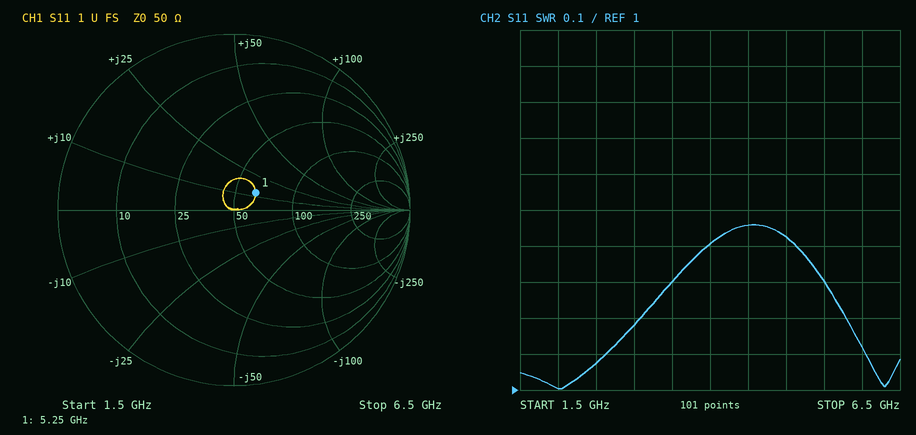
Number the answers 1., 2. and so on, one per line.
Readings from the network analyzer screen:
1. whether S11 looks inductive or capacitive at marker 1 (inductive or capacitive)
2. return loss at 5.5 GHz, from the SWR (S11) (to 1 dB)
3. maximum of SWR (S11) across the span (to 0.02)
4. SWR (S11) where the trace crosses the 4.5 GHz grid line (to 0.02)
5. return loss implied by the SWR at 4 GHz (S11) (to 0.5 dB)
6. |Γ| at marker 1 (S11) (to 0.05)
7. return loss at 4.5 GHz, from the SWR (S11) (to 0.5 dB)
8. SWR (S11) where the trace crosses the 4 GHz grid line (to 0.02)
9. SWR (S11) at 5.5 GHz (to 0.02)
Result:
1. inductive
2. 18 dB
3. 1.46
4. 1.46
5. 15.5 dB
6. 0.15
7. 14.5 dB
8. 1.40
9. 1.30
